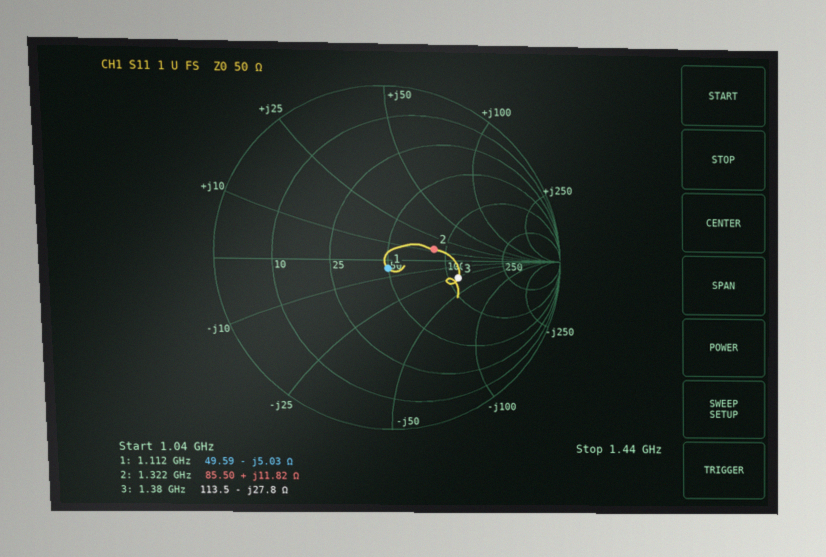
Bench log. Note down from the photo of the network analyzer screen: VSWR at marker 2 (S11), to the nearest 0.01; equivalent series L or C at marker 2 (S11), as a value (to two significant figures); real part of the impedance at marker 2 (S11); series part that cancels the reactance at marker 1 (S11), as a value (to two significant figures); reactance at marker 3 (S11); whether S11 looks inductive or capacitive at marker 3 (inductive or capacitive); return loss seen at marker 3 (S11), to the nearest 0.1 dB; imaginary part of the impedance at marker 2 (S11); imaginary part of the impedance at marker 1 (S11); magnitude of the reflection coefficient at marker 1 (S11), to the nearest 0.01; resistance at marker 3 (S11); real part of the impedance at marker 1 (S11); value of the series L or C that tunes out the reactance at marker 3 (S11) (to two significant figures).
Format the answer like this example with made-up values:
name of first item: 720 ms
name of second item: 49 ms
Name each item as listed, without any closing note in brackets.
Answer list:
VSWR at marker 2 (S11), to the nearest 0.01: 1.76
equivalent series L or C at marker 2 (S11), as a value: 1.4 nH
real part of the impedance at marker 2: 85.50 Ω
series part that cancels the reactance at marker 1 (S11), as a value: 720 pH
reactance at marker 3: -27.8 Ω
whether S11 looks inductive or capacitive at marker 3: capacitive
return loss seen at marker 3 (S11), to the nearest 0.1 dB: 7.6 dB
imaginary part of the impedance at marker 2: +11.82 Ω
imaginary part of the impedance at marker 1: -5.03 Ω
magnitude of the reflection coefficient at marker 1 (S11), to the nearest 0.01: 0.05
resistance at marker 3: 113.5 Ω
real part of the impedance at marker 1: 49.59 Ω
value of the series L or C that tunes out the reactance at marker 3 (S11): 3.2 nH
